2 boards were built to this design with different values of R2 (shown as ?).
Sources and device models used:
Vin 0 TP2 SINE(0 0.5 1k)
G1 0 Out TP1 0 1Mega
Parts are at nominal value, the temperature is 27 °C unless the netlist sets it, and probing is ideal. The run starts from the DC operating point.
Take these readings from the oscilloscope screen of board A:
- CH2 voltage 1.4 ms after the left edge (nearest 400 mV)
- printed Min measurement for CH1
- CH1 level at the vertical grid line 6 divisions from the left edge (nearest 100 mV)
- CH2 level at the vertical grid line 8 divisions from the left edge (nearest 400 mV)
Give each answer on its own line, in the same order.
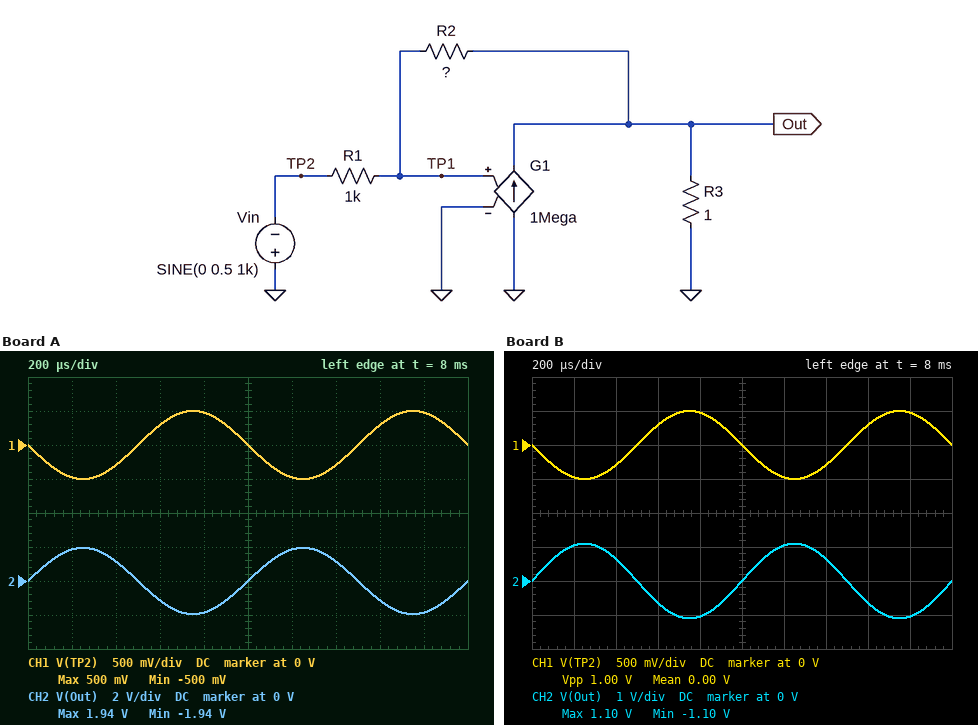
1.2 V
-500 mV
-500 mV
-1.2 V
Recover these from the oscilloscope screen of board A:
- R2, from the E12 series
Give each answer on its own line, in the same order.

3.9 kΩ
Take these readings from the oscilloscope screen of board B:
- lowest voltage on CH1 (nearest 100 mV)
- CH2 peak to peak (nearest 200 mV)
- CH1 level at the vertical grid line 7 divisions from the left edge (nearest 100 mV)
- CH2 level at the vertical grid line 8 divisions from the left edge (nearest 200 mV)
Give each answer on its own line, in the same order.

-500 mV
2.2 V
-300 mV
-600 mV
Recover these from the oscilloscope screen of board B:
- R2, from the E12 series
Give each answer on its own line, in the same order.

2.2 kΩ
